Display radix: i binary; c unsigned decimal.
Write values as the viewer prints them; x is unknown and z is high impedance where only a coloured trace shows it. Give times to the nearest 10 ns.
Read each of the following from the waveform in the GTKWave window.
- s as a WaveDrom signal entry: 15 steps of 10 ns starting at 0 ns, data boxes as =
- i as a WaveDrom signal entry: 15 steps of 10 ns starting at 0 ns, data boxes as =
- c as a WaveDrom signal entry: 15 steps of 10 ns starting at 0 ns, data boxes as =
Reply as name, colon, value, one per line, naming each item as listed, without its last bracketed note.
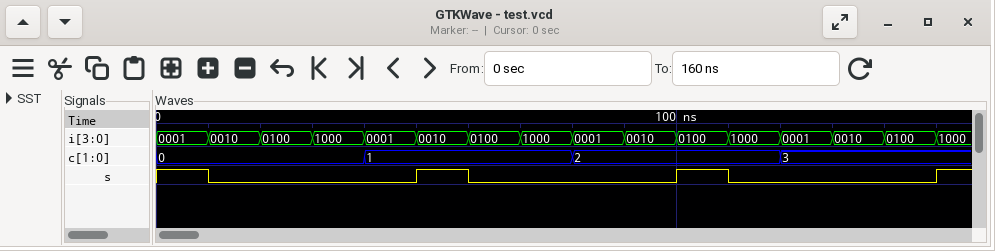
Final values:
s as a WaveDrom signal entry: 15 steps of 10 ns starting at 0 ns, data boxes as =: {name: 's', wave: '10...10...10...'}
i as a WaveDrom signal entry: 15 steps of 10 ns starting at 0 ns, data boxes as =: {name: 'i', wave: '===============', data: '0001 0010 0100 1000 0001 0010 0100 1000 0001 0010 0100 1000 0001 0010 0100'}
c as a WaveDrom signal entry: 15 steps of 10 ns starting at 0 ns, data boxes as =: {name: 'c', wave: '=...=...=...=..', data: '0 1 2 3'}
